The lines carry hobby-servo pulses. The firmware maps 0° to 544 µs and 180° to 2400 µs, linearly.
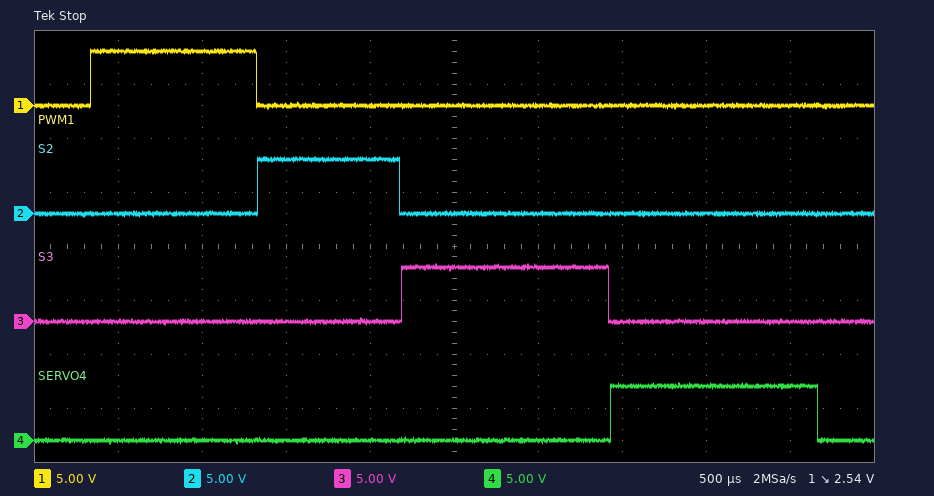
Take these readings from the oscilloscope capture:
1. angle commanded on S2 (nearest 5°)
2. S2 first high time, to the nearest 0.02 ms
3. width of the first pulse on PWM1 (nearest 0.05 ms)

30°
0.84 ms
1.00 ms
